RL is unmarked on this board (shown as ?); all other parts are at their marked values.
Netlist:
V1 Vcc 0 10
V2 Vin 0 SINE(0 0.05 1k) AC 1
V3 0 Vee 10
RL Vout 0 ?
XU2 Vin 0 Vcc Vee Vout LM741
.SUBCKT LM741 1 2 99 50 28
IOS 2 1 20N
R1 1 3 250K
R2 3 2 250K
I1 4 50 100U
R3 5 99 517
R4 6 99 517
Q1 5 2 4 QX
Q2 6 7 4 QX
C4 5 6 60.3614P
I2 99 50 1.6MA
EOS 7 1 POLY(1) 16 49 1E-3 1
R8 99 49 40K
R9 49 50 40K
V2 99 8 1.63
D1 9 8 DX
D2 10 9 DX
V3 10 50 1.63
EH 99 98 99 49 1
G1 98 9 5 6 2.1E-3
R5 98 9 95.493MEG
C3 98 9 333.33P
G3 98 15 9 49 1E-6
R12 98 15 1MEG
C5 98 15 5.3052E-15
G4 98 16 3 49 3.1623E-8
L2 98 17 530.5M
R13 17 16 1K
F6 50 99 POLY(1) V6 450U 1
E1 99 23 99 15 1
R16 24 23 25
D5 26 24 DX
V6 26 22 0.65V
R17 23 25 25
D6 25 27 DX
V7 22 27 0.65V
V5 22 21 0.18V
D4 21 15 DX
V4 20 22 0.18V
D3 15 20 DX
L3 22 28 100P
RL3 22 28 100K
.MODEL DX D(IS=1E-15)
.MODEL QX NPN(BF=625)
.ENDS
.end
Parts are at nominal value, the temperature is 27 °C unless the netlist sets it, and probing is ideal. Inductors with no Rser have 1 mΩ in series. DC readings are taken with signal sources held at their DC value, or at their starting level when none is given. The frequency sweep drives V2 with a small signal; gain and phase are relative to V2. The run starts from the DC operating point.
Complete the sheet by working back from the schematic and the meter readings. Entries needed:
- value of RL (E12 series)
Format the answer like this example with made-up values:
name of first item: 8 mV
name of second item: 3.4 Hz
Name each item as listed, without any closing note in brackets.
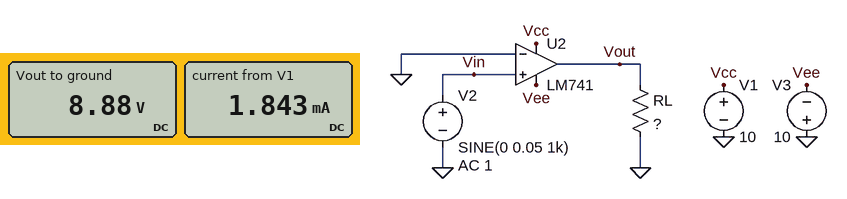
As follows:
value of RL: 27 kΩ
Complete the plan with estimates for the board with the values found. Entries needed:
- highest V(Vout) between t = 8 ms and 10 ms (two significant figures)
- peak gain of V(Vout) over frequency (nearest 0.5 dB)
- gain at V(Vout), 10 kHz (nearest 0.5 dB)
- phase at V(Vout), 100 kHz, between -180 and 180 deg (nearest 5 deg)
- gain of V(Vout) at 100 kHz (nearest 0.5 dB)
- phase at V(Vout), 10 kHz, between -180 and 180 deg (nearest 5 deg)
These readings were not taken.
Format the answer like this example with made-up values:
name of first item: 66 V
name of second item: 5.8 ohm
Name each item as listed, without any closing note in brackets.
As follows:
highest V(Vout) between t = 8 ms and 10 ms: 9.0 V
peak gain of V(Vout) over frequency: 28.5 dB
gain at V(Vout), 10 kHz: 28.5 dB
phase at V(Vout), 100 kHz, between -180 and 180 deg: -70 deg
gain of V(Vout) at 100 kHz: 19.5 dB
phase at V(Vout), 10 kHz, between -180 and 180 deg: -15 deg
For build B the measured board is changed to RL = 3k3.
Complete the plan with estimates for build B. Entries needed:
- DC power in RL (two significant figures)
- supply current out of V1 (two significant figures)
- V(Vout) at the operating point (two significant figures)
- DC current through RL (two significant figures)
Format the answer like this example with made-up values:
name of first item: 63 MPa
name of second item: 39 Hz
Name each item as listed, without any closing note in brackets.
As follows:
DC power in RL: 23 mW
supply current out of V1: 4.2 mA
V(Vout) at the operating point: 8.8 V
DC current through RL: 2.7 mA
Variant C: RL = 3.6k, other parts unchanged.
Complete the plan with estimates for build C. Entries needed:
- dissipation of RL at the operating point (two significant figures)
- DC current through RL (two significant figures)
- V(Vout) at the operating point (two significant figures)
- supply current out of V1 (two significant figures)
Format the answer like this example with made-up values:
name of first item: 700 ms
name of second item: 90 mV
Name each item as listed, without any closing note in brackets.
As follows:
dissipation of RL at the operating point: 21 mW
DC current through RL: 2.4 mA
V(Vout) at the operating point: 8.8 V
supply current out of V1: 3.9 mA
